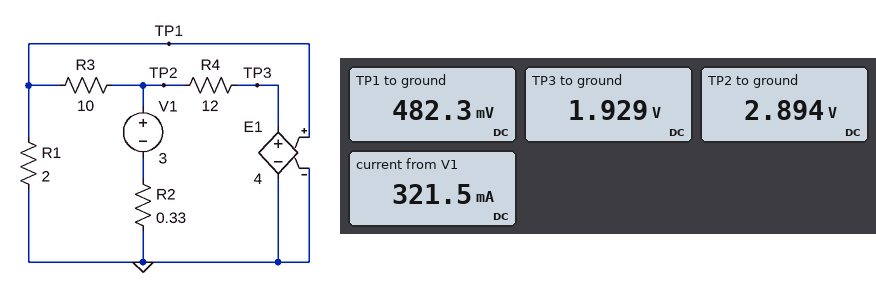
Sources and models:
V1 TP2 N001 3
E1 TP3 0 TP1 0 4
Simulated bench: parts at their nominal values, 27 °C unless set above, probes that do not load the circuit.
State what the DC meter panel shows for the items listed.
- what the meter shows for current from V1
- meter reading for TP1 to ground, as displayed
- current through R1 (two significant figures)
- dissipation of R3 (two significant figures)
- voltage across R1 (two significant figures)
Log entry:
321.5 mA
482.3 mV
240 mA
580 mW
480 mV
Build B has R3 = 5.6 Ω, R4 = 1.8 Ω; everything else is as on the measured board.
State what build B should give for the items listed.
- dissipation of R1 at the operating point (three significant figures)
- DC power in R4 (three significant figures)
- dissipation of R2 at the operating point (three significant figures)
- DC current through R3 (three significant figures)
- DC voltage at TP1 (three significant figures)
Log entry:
292 mW
13.0 mW
29.1 mW
382 mA
764 mV
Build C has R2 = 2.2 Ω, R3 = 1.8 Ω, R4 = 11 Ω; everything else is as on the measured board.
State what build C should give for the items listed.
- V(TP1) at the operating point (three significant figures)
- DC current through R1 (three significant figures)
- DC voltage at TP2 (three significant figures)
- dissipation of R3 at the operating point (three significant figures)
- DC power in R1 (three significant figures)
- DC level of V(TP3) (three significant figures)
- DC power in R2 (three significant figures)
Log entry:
1.16 V
581 mA
2.21 V
608 mW
676 mW
4.65 V
284 mW
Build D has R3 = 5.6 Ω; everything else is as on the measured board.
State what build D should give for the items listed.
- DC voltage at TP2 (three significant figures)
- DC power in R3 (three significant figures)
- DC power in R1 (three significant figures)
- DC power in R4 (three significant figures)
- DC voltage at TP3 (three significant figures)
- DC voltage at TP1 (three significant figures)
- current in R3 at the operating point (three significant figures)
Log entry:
2.88 V
804 mW
287 mW
1.91 mW
3.03 V
758 mV
379 mA
